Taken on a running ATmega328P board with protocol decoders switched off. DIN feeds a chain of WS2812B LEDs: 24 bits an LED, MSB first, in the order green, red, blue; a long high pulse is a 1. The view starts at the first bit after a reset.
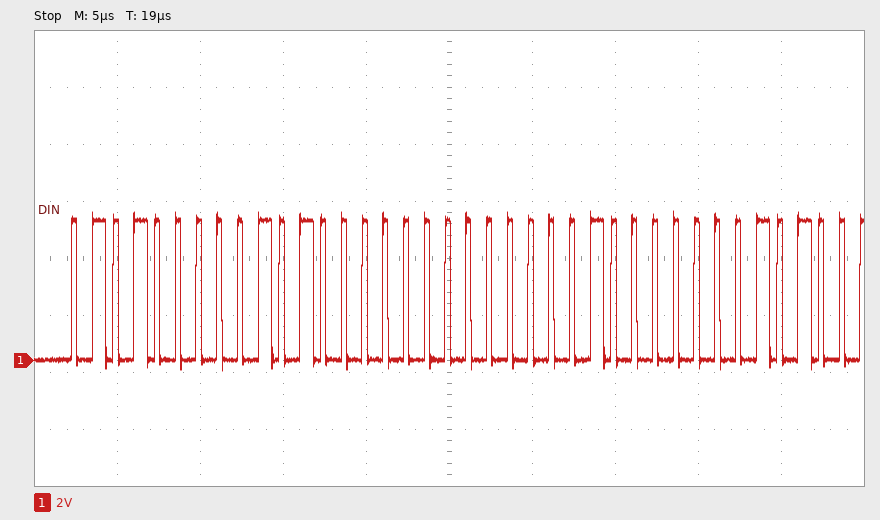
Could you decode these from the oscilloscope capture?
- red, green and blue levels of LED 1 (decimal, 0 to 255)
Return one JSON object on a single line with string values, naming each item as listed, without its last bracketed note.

{"red, green and blue levels of LED 1": "80, 80, 0"}
